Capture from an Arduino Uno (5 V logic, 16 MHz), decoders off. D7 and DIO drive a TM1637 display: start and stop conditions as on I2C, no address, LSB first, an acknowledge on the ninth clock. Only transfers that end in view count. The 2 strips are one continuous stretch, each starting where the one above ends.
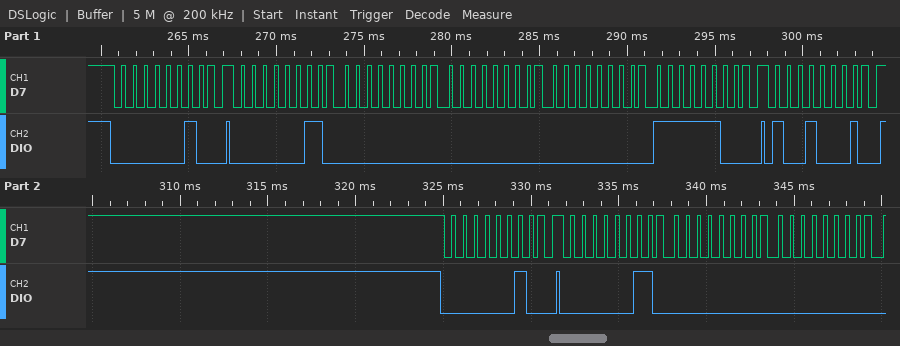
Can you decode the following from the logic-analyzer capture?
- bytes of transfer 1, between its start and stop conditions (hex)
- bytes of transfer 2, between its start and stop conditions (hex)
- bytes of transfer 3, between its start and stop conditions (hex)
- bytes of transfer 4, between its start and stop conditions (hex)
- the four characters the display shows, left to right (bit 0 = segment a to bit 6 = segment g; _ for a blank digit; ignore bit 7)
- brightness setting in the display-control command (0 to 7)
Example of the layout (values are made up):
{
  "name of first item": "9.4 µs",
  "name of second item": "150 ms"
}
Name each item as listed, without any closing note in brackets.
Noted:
{
  "bytes of transfer 1, between its start and stop conditions": "40",
  "bytes of transfer 2, between its start and stop conditions": "C0 00 00 00 3F",
  "bytes of transfer 3, between its start and stop conditions": "89",
  "bytes of transfer 4, between its start and stop conditions": "40",
  "the four characters the display shows, left to right": "___0",
  "brightness setting in the display-control command": "1"
}
